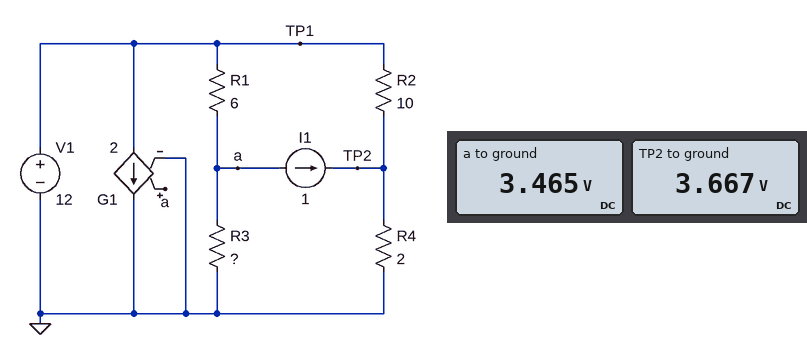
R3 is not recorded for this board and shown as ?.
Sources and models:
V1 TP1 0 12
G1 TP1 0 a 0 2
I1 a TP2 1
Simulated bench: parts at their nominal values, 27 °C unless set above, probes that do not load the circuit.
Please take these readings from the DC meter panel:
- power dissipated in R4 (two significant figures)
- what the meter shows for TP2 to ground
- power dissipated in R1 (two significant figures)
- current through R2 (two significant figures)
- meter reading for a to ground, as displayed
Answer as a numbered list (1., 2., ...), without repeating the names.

1. 6.7 W
2. 3.667 V
3. 12 W
4. 830 mA
5. 3.465 V
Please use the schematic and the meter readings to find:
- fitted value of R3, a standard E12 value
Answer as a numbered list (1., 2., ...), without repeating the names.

1. 8.2 Ω
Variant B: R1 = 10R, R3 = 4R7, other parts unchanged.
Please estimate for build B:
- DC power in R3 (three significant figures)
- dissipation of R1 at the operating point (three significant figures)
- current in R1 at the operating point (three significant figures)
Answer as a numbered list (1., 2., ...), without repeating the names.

1. 87.0 mW
2. 12.9 W
3. 1.14 A
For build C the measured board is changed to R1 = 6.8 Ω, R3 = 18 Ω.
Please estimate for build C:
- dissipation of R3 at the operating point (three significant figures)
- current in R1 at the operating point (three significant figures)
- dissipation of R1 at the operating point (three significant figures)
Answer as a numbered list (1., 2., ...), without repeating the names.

1. 791 mW
2. 1.21 A
3. 9.95 W
